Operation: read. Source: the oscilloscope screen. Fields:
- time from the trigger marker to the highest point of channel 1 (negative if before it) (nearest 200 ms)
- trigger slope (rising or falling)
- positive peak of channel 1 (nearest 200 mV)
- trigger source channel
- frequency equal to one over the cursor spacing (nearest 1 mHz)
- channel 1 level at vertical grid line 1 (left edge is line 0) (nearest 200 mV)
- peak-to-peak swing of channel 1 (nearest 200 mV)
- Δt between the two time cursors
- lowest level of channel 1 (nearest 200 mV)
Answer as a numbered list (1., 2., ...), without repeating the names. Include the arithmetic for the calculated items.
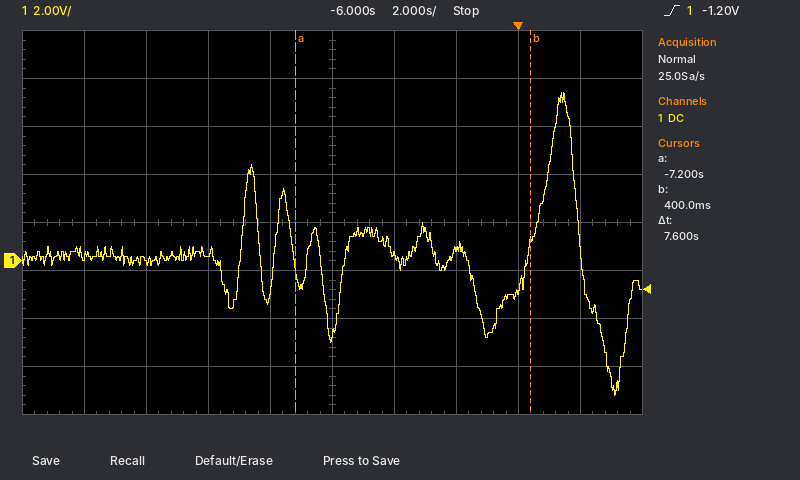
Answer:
1. +1.4 s
2. rising
3. 7.0 V
4. channel 1
5. 1 / 7.6 s ≈ 132 mHz
6. 200 mV
7. 7.0 V − (-5.6 V) = 12.6 V
8. 7.6 s
9. -5.6 V
